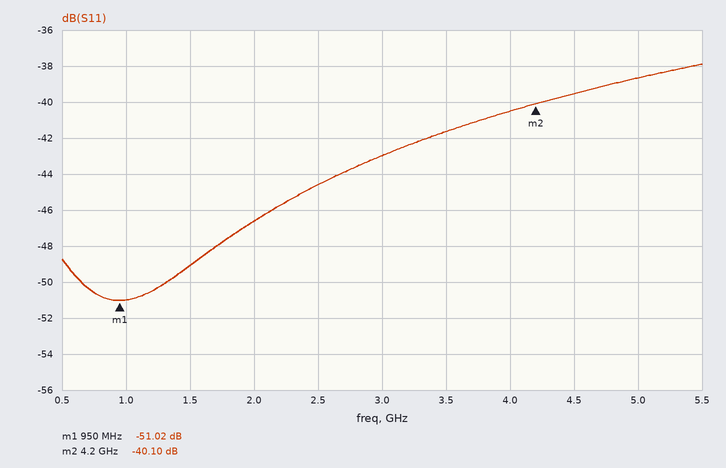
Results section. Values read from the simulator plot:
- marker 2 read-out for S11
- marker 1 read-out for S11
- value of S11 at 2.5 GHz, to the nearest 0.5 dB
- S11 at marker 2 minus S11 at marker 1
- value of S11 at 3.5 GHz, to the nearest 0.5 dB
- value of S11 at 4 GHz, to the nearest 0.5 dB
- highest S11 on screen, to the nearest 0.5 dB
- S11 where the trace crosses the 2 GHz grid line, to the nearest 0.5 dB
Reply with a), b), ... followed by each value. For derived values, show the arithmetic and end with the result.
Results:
a) -40.10 dB
b) -51.02 dB
c) -44.5 dB
d) -40.1 − (-51.02) = 10.92 dB
e) -41.5 dB
f) -40.5 dB
g) -38.0 dB
h) -46.5 dB
